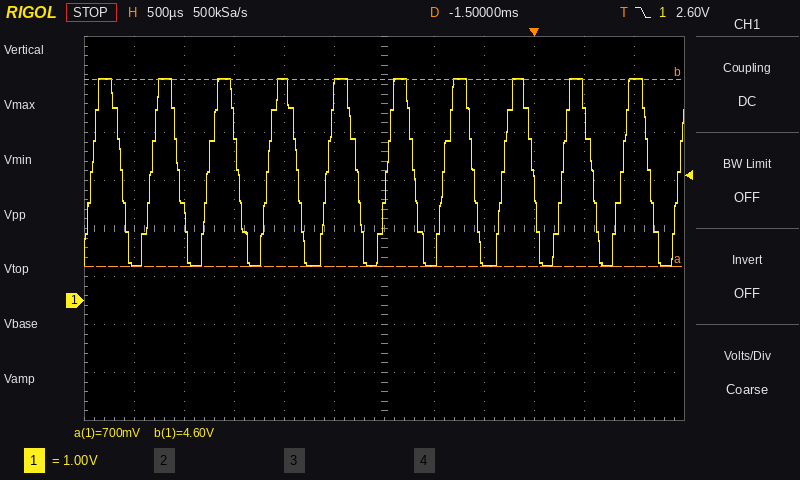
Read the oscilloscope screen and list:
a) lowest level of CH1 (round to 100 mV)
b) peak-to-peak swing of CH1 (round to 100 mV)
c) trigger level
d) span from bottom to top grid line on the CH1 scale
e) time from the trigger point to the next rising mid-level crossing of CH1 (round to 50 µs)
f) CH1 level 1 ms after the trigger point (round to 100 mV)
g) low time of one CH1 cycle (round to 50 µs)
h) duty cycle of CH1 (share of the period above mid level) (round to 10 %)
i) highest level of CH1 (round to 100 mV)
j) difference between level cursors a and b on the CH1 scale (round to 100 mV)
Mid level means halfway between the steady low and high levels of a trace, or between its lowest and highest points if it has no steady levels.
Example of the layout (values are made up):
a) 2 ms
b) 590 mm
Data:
a) 700 mV
b) 3.9 V
c) 2.60 V
d) 8 V
e) 300 µs
f) 4.6 V
g) 300 µs
h) 50 %
i) 4.6 V
j) 3.9 V
